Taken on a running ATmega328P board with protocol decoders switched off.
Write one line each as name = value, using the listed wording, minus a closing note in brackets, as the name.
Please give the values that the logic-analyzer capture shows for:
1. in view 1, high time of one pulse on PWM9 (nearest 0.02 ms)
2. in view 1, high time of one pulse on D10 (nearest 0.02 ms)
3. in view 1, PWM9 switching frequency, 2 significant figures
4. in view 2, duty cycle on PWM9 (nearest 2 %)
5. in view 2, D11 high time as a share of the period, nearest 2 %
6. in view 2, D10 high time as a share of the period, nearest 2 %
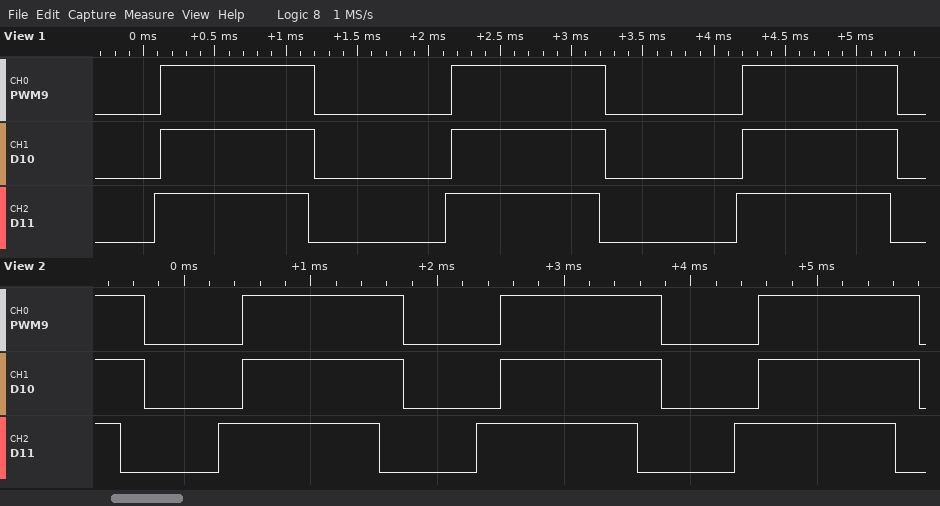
in view 1, high time of one pulse on PWM9 = 1.08 ms
in view 1, high time of one pulse on D10 = 1.08 ms
in view 1, PWM9 switching frequency, 2 significant figures = 490 Hz
in view 2, duty cycle on PWM9 = 62 %
in view 2, D11 high time as a share of the period, nearest 2 % = 62 %
in view 2, D10 high time as a share of the period, nearest 2 % = 62 %
